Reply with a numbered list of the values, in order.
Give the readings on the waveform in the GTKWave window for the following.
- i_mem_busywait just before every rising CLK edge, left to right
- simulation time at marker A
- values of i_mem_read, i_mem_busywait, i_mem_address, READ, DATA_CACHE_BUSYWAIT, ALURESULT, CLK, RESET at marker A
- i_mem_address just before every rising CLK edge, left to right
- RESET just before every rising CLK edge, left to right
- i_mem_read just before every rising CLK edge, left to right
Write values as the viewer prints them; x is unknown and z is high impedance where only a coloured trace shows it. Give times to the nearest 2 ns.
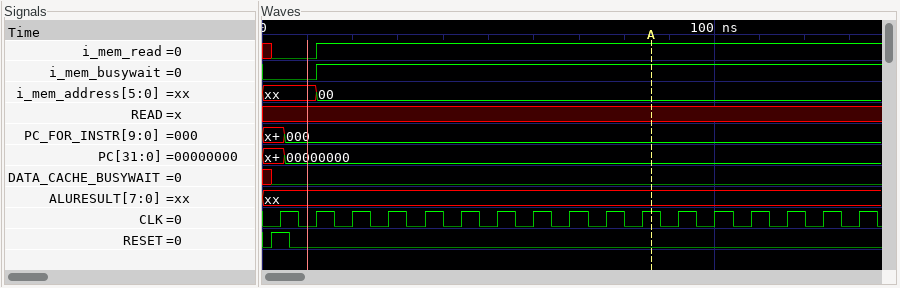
1. 0 0 1 1 1 1 1 1 1 1 1 1 1 1 1 1 1
2. 86 ns
3. i_mem_read=1, i_mem_busywait=1, i_mem_address=00, READ=x, DATA_CACHE_BUSYWAIT=0, ALURESULT=xx, CLK=1, RESET=0
4. xx, xx, 00, 00, 00, 00, 00, 00, 00, 00, 00, 00, 00, 00, 00, 00, 00
5. 1 0 0 0 0 0 0 0 0 0 0 0 0 0 0 0 0
6. 0 0 1 1 1 1 1 1 1 1 1 1 1 1 1 1 1
